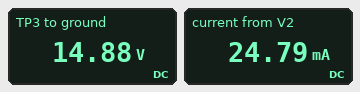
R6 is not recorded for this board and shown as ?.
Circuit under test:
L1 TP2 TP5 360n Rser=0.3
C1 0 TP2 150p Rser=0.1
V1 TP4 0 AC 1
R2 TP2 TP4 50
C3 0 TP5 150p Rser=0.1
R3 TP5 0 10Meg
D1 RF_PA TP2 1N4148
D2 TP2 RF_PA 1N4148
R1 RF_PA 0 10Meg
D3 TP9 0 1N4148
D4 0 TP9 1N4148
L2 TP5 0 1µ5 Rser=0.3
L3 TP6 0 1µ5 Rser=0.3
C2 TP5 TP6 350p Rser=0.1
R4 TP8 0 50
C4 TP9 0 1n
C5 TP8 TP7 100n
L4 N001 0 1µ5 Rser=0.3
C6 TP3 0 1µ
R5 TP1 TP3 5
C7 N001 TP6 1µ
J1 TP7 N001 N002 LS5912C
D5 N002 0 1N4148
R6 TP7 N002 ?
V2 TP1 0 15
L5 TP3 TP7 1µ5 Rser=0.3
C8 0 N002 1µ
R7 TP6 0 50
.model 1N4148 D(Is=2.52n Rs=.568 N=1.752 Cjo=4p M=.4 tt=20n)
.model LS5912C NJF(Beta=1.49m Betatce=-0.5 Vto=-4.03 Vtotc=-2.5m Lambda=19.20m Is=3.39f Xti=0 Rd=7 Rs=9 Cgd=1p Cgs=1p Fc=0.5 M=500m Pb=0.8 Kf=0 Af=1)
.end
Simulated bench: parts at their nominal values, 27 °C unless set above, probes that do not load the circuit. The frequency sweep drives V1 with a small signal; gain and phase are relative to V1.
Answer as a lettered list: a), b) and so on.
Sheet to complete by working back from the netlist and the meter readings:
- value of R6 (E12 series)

a) 2.2 kΩ
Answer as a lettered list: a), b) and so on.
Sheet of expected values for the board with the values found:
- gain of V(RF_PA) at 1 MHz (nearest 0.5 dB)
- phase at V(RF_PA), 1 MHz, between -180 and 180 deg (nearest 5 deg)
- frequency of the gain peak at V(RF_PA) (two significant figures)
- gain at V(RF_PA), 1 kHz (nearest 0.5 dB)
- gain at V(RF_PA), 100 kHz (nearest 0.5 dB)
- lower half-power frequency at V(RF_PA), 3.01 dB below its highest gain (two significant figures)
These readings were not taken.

a) -12.5 dB
b) 75 deg
c) 4.5 MHz
d) -43.5 dB
e) -31.5 dB
f) 2.8 MHz
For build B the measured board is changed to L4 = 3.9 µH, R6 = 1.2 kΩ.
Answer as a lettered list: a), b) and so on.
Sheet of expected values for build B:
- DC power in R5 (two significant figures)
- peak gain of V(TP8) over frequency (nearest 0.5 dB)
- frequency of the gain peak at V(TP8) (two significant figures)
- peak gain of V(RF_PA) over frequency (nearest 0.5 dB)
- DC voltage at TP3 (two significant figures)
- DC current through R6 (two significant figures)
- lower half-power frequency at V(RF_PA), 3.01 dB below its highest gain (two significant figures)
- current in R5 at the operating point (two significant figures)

a) 4.5 mW
b) -12.5 dB
c) 22 MHz
d) -1.0 dB
e) 15 V
f) 12 mA
g) 2.7 MHz
h) 30 mA
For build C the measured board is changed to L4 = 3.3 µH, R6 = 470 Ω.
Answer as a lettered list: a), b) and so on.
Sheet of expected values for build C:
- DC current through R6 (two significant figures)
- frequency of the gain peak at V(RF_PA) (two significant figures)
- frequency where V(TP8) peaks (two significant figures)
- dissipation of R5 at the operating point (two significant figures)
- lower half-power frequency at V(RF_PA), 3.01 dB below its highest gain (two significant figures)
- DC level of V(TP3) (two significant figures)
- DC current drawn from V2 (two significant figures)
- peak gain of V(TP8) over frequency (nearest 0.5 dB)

a) 30 mA
b) 4.4 MHz
c) 22 MHz
d) 11 mW
e) 2.7 MHz
f) 15 V
g) 48 mA
h) -13.0 dB
